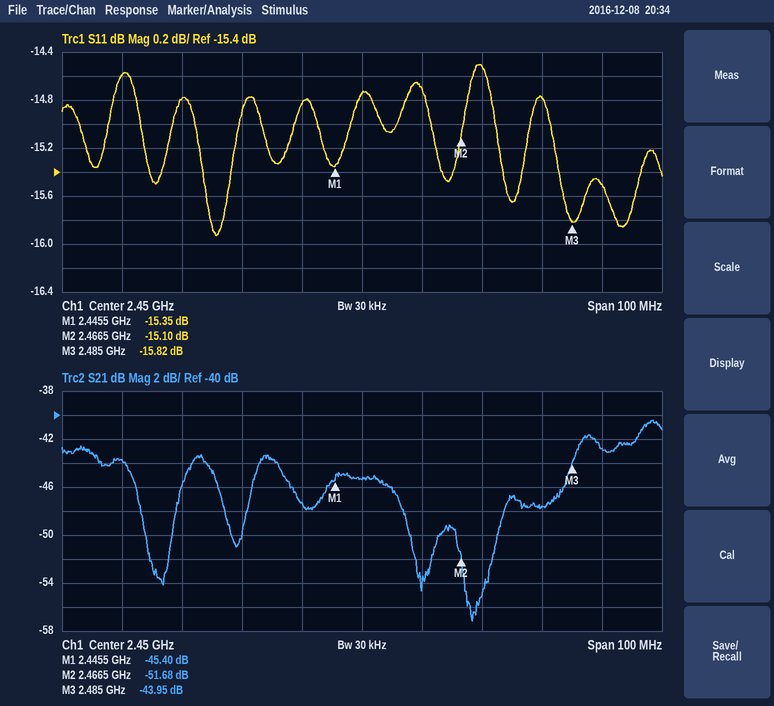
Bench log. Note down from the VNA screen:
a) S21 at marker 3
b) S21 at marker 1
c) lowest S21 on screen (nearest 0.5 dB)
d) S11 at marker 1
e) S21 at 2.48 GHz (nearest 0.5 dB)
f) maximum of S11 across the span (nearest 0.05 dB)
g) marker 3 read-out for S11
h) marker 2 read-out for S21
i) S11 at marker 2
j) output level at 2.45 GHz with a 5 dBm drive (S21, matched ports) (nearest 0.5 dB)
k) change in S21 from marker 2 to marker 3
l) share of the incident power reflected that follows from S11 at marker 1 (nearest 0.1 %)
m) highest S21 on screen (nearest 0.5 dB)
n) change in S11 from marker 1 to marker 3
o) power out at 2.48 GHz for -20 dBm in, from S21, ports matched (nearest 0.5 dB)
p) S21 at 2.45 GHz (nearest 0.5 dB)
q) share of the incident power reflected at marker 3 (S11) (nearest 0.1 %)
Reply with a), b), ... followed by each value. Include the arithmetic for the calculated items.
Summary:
a) -43.95 dB
b) -45.40 dB
c) -57.0 dB
d) -15.35 dB
e) -47.5 dB
f) -14.50 dB
g) -15.82 dB
h) -51.68 dB
i) -15.10 dB
j) 5 dBm + (-45.5 dB) = -40.5 dBm
k) -43.95 − (-51.68) = 7.73 dB
l) 10^(-15.35/10) ≈ 2.9 %
m) -40.5 dB
n) -15.82 − (-15.35) = -0.47 dB
o) -20 dBm + (-47.5 dB) = -67.5 dBm
p) -45.5 dB
q) 10^(-15.82/10) ≈ 2.6 %
